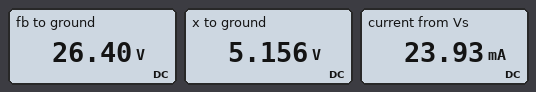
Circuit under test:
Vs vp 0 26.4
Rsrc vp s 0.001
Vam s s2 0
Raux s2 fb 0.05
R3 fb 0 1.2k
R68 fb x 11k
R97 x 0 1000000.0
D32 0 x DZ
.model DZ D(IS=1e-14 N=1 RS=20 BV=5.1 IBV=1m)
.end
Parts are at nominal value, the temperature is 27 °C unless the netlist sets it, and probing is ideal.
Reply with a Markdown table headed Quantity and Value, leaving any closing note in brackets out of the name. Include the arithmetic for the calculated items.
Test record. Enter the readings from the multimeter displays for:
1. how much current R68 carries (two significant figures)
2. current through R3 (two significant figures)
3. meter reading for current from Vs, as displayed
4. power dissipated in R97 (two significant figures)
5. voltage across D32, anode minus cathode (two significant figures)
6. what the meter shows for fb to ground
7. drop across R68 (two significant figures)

| Quantity | Value |
|---|---|
| how much current R68 carries | (26.4 V - 5.156 V) / 11 kΩ = 1.9 mA |
| current through R3 | (26.4 V) / 1.2 kΩ = 22 mA |
| meter reading for current from Vs, as displayed | 23.93 mA |
| power dissipated in R97 | (5.156 V)^2 / 1 MΩ = 27 µW |
| voltage across D32, anode minus cathode | 0 V - 5.156 V = -5.2 V |
| what the meter shows for fb to ground | 26.40 V |
| drop across R68 | 26.4 V - 5.156 V = 21 V |
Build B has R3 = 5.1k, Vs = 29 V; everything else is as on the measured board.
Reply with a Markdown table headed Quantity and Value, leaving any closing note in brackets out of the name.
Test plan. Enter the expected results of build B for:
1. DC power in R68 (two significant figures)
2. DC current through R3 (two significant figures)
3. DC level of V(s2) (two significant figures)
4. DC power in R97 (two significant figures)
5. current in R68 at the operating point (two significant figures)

| Quantity | Value |
|---|---|
| DC power in R68 | 52 mW |
| DC current through R3 | 5.7 mA |
| DC level of V(s2) | 29 V |
| DC power in R97 | 27 µW |
| current in R68 at the operating point | 2.2 mA |
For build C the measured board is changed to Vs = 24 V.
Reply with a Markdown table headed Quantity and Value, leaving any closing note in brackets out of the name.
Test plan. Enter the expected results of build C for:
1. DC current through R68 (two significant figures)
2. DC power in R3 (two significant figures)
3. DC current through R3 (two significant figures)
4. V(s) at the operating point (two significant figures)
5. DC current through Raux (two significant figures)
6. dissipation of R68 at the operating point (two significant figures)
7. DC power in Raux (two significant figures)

| Quantity | Value |
|---|---|
| DC current through R68 | 1.7 mA |
| DC power in R3 | 480 mW |
| DC current through R3 | 20 mA |
| V(s) at the operating point | 24 V |
| DC current through Raux | 22 mA |
| dissipation of R68 at the operating point | 32 mW |
| DC power in Raux | 24 µW |
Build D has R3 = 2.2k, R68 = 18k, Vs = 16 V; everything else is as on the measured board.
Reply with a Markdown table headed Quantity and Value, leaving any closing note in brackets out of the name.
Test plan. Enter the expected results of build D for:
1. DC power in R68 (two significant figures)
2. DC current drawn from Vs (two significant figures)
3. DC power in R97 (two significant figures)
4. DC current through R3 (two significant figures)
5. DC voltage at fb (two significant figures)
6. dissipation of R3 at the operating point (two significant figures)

| Quantity | Value |
|---|---|
| DC power in R68 | 6.6 mW |
| DC current drawn from Vs | 7.9 mA |
| DC power in R97 | 26 µW |
| DC current through R3 | 7.3 mA |
| DC voltage at fb | 16 V |
| dissipation of R3 at the operating point | 120 mW |
